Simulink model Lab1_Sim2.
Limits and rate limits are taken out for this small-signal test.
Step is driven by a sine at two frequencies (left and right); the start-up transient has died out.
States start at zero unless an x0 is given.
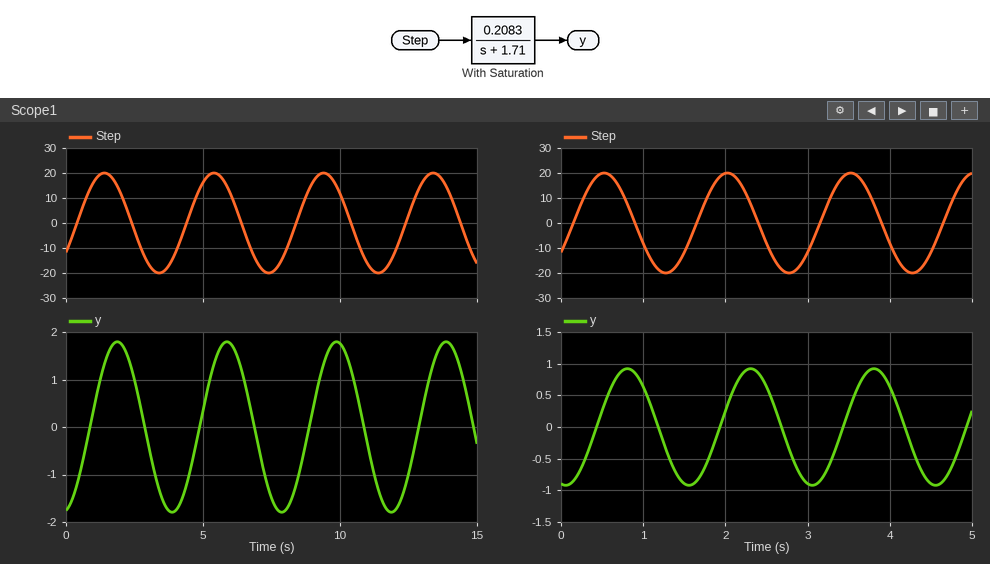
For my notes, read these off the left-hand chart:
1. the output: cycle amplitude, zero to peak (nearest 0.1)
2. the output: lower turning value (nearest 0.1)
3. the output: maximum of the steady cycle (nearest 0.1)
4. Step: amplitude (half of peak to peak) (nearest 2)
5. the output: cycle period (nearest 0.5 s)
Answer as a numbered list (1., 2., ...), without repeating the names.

1. 1.8
2. -1.8
3. 1.8
4. 20
5. 4.0 s
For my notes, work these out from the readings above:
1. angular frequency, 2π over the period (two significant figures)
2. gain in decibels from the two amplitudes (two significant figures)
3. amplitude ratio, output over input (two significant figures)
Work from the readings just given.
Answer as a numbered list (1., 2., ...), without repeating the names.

1. 1.6 rad/s
2. -21 dB
3. 0.090
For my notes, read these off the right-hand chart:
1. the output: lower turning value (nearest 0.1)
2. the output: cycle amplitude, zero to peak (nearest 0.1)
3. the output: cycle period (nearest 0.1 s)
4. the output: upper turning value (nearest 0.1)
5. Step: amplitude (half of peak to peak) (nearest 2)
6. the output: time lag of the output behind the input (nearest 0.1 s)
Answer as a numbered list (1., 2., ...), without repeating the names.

1. -0.9
2. 0.9
3. 1.5 s
4. 0.9
5. 20
6. 0.3 s
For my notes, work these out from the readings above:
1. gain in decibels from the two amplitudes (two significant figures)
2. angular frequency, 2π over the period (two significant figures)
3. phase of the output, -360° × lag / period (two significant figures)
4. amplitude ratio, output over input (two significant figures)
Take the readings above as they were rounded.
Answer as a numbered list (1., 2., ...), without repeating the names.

1. -27 dB
2. 4.2 rad/s
3. -72°
4. 0.045
